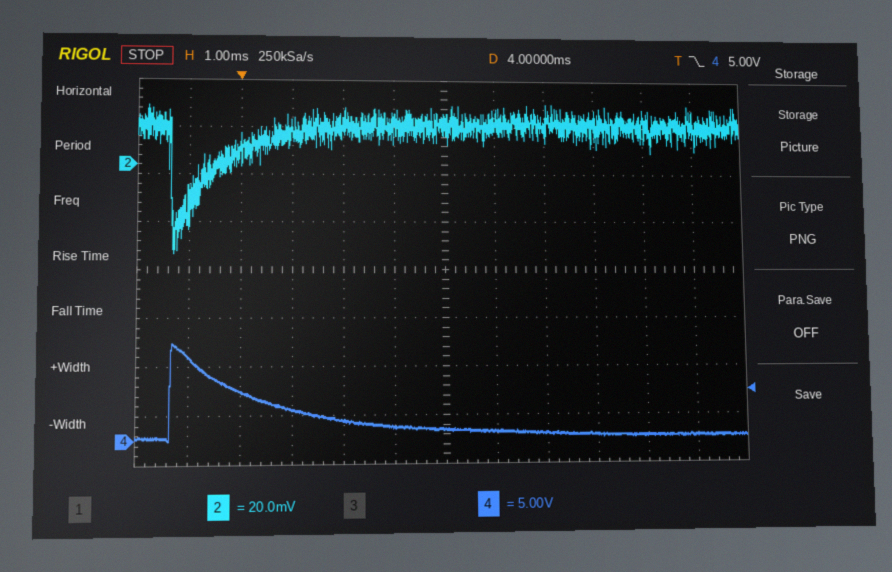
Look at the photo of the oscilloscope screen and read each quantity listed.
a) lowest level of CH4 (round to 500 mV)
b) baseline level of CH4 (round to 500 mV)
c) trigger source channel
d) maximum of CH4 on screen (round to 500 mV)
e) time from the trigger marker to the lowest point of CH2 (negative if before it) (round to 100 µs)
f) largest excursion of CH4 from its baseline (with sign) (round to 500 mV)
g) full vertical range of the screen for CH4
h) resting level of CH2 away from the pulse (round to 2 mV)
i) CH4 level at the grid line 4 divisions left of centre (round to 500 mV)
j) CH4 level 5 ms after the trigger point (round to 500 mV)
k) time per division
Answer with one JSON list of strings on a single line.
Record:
["0.0 V", "500 mV", "CH4", "10.0 V", "-1.3 ms", "+9.5 V", "40 V", "16 mV", "5.0 V", "1.0 V", "1 ms"]
